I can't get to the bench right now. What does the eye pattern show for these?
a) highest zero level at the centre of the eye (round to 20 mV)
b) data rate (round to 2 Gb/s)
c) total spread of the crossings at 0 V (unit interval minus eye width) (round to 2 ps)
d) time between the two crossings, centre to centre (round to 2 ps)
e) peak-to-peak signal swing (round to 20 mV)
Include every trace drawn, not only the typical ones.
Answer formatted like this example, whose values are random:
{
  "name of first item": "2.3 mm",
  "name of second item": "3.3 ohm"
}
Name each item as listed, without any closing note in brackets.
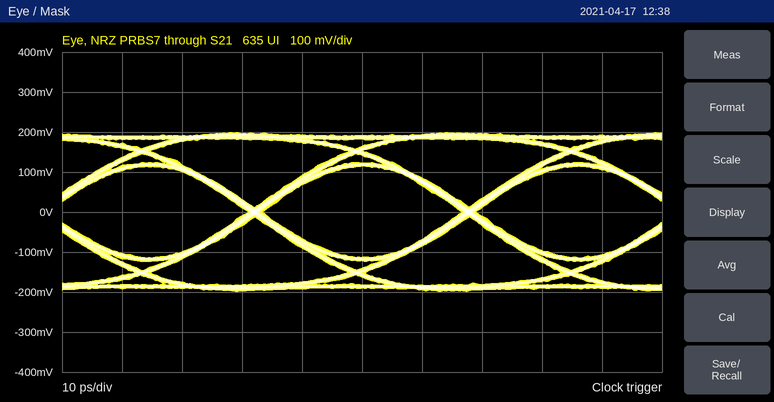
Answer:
{
  "highest zero level at the centre of the eye": "-120 mV",
  "data rate": "28 Gb/s",
  "total spread of the crossings at 0 V (unit interval minus eye width)": "2 ps",
  "time between the two crossings, centre to centre": "36 ps",
  "peak-to-peak signal swing": "400 mV"
}
